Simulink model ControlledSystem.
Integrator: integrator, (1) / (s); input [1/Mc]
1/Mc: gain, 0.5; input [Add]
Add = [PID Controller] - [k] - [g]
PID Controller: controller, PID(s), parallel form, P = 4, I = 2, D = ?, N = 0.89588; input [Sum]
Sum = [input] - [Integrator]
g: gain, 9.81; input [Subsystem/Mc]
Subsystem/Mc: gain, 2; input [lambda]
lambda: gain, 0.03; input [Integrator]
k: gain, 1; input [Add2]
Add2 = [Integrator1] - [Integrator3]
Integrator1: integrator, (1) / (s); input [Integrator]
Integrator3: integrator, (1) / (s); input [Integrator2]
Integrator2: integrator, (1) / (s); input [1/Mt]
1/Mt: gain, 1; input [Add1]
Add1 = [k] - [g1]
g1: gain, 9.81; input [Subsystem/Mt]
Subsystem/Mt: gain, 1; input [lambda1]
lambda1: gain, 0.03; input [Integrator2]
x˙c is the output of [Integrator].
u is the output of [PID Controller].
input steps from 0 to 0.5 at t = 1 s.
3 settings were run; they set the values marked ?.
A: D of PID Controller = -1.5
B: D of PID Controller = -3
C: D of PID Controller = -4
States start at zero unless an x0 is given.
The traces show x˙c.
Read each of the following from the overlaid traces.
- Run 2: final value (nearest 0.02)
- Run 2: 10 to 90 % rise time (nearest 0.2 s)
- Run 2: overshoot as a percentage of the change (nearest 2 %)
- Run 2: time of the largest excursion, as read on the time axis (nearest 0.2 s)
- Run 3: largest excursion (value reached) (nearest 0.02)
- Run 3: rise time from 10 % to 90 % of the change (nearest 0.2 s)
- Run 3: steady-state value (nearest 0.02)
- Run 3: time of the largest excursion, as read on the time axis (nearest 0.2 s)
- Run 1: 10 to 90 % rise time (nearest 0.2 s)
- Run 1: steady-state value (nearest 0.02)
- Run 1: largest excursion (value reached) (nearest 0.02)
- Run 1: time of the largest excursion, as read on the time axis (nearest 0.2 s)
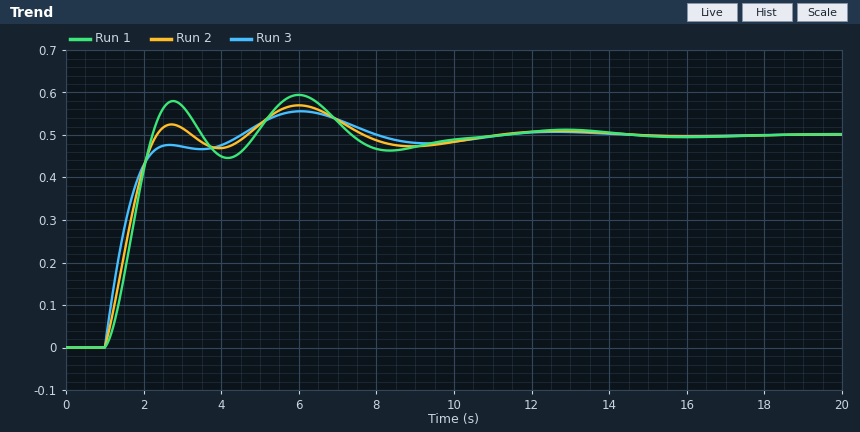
0.50
1.0 s
14 %
6.0 s
0.56
1.0 s
0.50
6.0 s
0.8 s
0.50
0.60
6.0 s
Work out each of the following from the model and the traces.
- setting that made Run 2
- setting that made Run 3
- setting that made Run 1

B
A
C
